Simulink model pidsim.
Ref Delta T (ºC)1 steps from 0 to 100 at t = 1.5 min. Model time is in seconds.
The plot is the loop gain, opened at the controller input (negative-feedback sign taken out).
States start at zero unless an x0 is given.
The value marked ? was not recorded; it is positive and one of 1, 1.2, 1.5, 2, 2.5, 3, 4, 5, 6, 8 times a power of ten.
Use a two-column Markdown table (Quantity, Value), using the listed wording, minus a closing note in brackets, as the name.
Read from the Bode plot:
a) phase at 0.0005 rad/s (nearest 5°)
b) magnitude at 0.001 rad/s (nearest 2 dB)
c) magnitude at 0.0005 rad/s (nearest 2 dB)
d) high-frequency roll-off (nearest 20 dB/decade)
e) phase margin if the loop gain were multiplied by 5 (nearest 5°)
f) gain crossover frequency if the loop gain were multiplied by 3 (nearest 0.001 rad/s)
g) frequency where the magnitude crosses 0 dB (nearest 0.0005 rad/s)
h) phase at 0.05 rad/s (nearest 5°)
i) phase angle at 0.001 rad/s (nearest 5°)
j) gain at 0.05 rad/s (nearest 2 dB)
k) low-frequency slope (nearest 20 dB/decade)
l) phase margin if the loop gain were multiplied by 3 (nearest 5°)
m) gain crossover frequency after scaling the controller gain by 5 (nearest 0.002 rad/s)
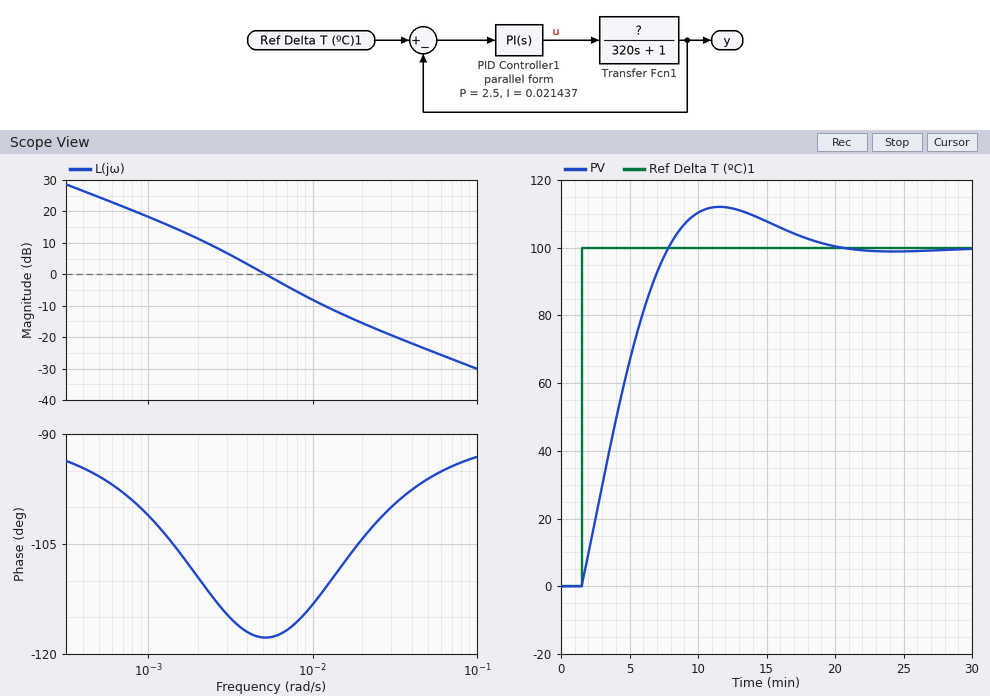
| Quantity | Value |
|---|---|
| phase at 0.0005 rad/s | -95° |
| magnitude at 0.001 rad/s | 18 dB |
| magnitude at 0.0005 rad/s | 24 dB |
| high-frequency roll-off | -20 dB/decade |
| phase margin if the loop gain were multiplied by 5 | 75° |
| gain crossover frequency if the loop gain were multiplied by 3 | 0.011 rad/s |
| frequency where the magnitude crosses 0 dB | 0.0050 rad/s |
| phase at 0.05 rad/s | -95° |
| phase angle at 0.001 rad/s | -100° |
| gain at 0.05 rad/s | -24 dB |
| low-frequency slope | -20 dB/decade |
| phase margin if the loop gain were multiplied by 3 | 70° |
| gain crossover frequency after scaling the controller gain by 5 | 0.018 rad/s |
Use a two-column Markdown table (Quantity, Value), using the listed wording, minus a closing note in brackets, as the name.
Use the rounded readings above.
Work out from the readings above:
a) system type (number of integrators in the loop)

| Quantity | Value |
|---|---|
| system type | 1 |
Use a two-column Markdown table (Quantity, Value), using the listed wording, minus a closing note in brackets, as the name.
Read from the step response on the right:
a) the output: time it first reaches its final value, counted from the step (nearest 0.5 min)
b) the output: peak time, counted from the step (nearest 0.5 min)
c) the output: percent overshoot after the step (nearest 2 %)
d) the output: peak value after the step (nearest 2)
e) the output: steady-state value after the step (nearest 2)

| Quantity | Value |
|---|---|
| the output: time it first reaches its final value, counted from the step | 6.5 min |
| the output: peak time, counted from the step | 10.0 min |
| the output: percent overshoot after the step | 12 % |
| the output: peak value after the step | 112 |
| the output: steady-state value after the step | 100 |
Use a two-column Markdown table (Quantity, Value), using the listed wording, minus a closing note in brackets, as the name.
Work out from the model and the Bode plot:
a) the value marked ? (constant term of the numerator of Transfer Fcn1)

| Quantity | Value |
|---|---|
| the value marked ? | 0.4 |
